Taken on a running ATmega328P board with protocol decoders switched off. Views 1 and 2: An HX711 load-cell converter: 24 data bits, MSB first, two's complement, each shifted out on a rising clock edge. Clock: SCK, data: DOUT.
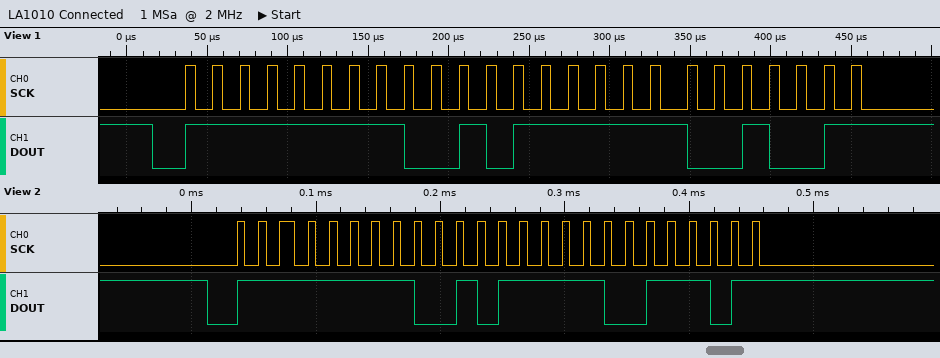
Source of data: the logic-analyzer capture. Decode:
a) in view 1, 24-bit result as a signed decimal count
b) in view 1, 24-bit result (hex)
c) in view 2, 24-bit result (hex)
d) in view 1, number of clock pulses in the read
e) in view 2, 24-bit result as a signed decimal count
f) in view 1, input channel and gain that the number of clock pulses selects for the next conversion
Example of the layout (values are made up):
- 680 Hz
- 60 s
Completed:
- -53303
- 0xFF2FC9
- 0xFF2F9D
- 25
- -53347
- channel A, gain 128
